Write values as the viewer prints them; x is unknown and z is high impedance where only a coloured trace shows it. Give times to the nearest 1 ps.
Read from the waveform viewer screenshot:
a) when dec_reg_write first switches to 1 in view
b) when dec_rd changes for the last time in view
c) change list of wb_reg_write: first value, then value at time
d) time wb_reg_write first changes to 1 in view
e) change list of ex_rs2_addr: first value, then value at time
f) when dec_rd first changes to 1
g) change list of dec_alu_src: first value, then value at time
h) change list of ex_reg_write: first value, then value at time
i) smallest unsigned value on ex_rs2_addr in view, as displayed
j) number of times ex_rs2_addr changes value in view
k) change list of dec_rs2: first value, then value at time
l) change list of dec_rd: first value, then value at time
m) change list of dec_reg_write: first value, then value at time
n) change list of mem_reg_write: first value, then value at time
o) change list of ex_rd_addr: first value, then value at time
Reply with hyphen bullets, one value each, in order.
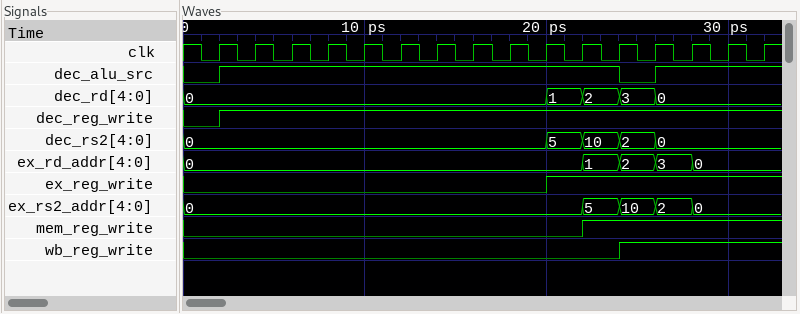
- 2 ps
- 26 ps
- 0, 1 at 24 ps
- 24 ps
- 0, 5 at 22 ps, 10 at 24 ps, 2 at 26 ps, 0 at 28 ps
- 20 ps
- 0, 1 at 2 ps, 0 at 24 ps, 1 at 26 ps
- 0, 1 at 20 ps
- 0
- 4
- 0, 5 at 20 ps, 10 at 22 ps, 2 at 24 ps, 0 at 26 ps
- 0, 1 at 20 ps, 2 at 22 ps, 3 at 24 ps, 0 at 26 ps
- 0, 1 at 2 ps
- 0, 1 at 22 ps
- 0, 1 at 22 ps, 2 at 24 ps, 3 at 26 ps, 0 at 28 ps
